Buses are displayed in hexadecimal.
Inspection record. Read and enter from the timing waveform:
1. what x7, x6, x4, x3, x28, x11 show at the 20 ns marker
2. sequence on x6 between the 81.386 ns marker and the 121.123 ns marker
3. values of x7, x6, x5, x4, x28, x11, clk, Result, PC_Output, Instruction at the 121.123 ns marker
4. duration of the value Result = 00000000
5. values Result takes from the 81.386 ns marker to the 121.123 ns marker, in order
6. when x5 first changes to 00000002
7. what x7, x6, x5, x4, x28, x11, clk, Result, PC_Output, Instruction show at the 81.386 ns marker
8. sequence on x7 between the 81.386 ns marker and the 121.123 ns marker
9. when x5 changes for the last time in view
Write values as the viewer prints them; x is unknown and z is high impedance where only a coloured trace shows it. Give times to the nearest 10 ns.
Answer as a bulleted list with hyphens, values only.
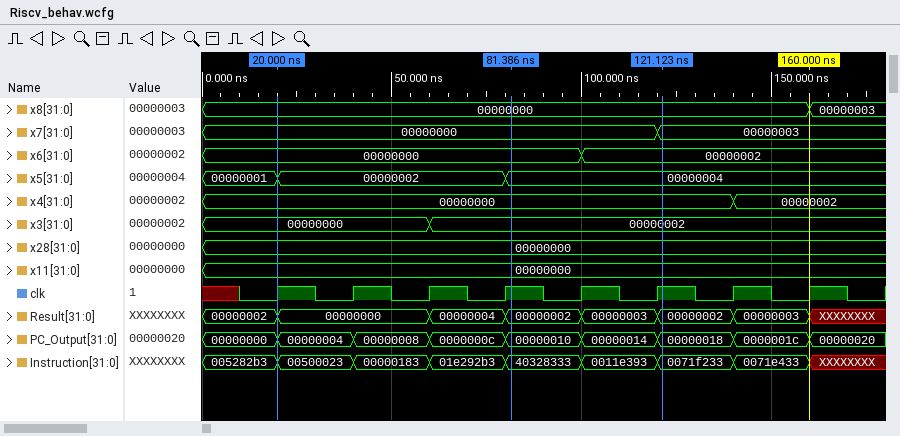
- x7=00000000, x6=00000000, x4=00000000, x3=00000000, x28=00000000, x11=00000000
- 00000000, 00000002
- x7=00000003, x6=00000002, x5=00000004, x4=00000000, x28=00000000, x11=00000000, clk=1, Result=00000002, PC_Output=00000018, Instruction=0071f233
- 40 ns
- 00000002, 00000003, 00000002
- 20 ns
- x7=00000000, x6=00000000, x5=00000004, x4=00000000, x28=00000000, x11=00000000, clk=1, Result=00000002, PC_Output=00000010, Instruction=40328333
- 00000000, 00000003
- 80 ns
